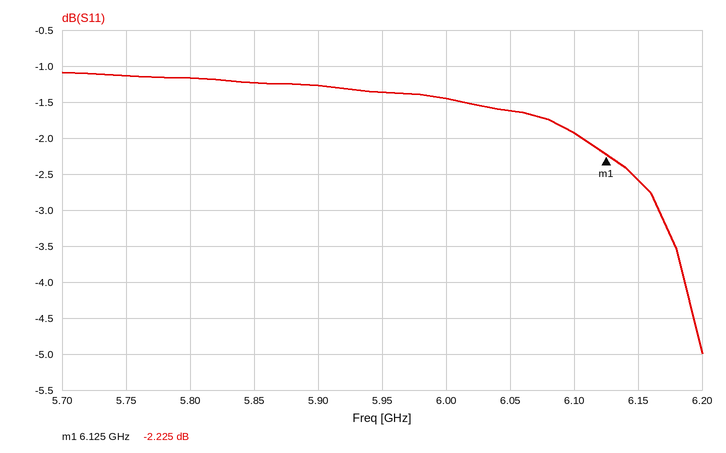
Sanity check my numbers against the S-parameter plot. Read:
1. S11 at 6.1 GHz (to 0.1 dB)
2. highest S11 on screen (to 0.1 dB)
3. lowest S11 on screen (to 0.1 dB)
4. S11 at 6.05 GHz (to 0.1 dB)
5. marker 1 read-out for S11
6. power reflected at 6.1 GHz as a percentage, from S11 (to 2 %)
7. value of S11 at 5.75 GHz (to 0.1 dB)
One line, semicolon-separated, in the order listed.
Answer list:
-1.9 dB; -1.1 dB; -5.0 dB; -1.6 dB; -2.225 dB; 64 %; -1.1 dB
